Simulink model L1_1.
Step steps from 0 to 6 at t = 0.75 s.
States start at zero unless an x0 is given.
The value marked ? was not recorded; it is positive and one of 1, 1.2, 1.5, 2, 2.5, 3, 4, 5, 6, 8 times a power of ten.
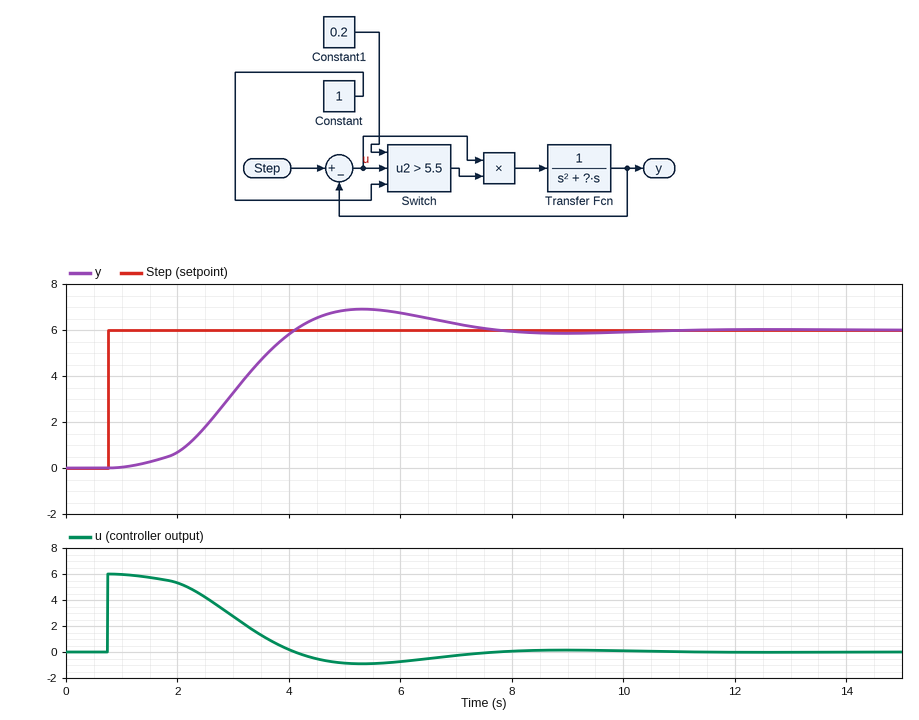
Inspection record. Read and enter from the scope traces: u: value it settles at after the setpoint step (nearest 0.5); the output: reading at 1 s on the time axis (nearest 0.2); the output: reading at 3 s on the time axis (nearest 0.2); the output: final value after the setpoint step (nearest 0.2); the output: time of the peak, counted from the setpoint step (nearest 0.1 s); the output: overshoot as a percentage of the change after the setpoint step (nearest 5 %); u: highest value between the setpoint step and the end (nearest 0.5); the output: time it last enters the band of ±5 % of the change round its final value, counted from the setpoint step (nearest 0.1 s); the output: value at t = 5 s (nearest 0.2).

0.0
0.0
3.2
6.0
4.6 s
15 %
6.0
6.2 s
6.8
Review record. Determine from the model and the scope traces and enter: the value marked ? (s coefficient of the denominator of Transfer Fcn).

1
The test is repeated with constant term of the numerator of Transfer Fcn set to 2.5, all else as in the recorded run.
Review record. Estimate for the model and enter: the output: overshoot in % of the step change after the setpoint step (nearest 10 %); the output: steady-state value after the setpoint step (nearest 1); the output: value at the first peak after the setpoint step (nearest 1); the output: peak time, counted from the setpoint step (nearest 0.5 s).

30 %
6
8
2.5 s
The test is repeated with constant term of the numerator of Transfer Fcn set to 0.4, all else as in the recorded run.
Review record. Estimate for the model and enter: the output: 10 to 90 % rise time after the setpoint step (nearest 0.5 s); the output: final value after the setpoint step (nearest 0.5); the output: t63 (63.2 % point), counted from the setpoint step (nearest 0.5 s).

4.0 s
6.0
4.5 s
